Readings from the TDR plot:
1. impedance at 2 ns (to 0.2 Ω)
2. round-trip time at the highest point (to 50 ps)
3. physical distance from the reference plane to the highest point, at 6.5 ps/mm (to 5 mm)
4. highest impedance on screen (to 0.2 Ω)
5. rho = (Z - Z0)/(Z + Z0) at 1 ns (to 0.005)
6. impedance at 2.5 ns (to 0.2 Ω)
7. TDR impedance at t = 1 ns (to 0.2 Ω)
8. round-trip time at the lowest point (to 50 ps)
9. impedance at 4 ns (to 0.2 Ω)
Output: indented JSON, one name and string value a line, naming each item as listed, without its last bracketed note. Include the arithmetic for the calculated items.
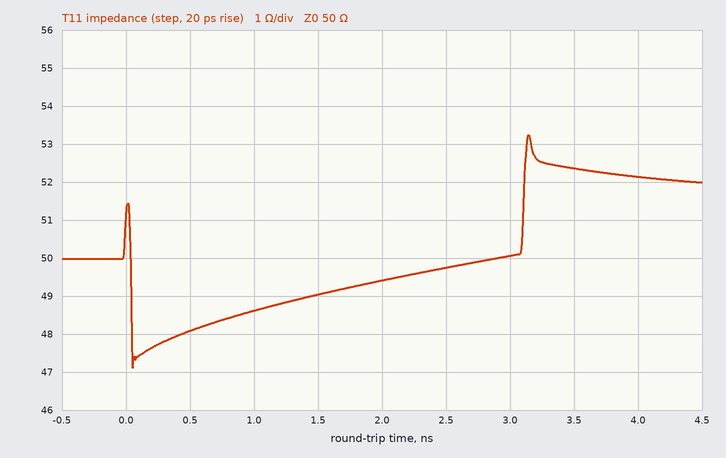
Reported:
{
  "impedance at 2 ns": "49.4 Ω",
  "round-trip time at the highest point": "3.15 ns",
  "physical distance from the reference plane to the highest point, at 6.5 ps/mm": "3.15 ns / 2 / 6.5 ps/mm ≈ 242 mm, so 240 mm to the nearest 5 mm",
  "highest impedance on screen": "53.2 Ω",
  "rho = (Z - Z0)/(Z + Z0) at 1 ns": "(48.6 − 50)/(48.6 + 50) ≈ -0.0142, so -0.015 to the nearest 0.005",
  "impedance at 2.5 ns": "49.8 Ω",
  "TDR impedance at t = 1 ns": "48.6 Ω",
  "round-trip time at the lowest point": "50 ps",
  "impedance at 4 ns": "52.2 Ω"
}
